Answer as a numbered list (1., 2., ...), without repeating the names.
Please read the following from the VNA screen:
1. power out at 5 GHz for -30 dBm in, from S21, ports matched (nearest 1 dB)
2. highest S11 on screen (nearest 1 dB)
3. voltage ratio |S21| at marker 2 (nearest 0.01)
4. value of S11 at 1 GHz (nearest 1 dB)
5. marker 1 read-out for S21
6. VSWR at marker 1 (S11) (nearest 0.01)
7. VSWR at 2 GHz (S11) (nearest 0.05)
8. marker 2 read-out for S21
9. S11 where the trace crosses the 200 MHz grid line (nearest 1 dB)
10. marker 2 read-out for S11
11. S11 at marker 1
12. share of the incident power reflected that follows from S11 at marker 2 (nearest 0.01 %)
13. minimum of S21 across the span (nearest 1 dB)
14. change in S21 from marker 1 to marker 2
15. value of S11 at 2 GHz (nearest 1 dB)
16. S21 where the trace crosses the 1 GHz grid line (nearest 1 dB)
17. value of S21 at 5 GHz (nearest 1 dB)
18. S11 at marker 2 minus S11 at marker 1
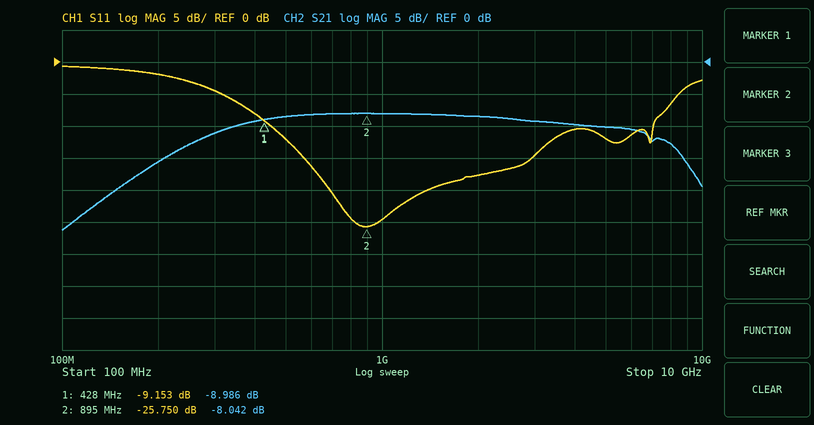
1. -40 dBm
2. -1 dB
3. 0.40
4. -25 dB
5. -8.986 dB
6. 2.07
7. 1.30
8. -8.042 dB
9. -2 dB
10. -25.750 dB
11. -9.153 dB
12. 0.27 %
13. -26 dB
14. 0.944 dB
15. -18 dB
16. -8 dB
17. -10 dB
18. -16.597 dB
